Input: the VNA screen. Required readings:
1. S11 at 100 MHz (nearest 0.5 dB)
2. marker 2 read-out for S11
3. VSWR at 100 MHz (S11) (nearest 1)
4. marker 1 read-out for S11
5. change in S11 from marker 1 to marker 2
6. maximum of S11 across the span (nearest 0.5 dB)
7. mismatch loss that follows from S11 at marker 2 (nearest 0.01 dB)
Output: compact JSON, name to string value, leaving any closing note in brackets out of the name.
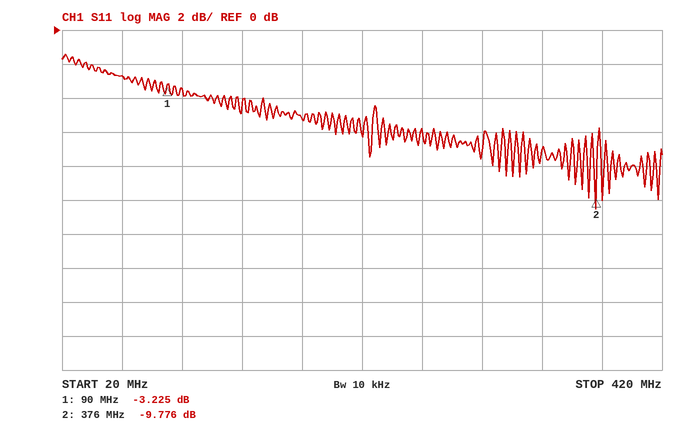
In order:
{"S11 at 100 MHz": "-3.5 dB", "marker 2 read-out for S11": "-9.776 dB", "VSWR at 100 MHz (S11)": "5", "marker 1 read-out for S11": "-3.225 dB", "change in S11 from marker 1 to marker 2": "-6.551 dB", "maximum of S11 across the span": "-1.5 dB", "mismatch loss that follows from S11 at marker 2": "0.48 dB"}
